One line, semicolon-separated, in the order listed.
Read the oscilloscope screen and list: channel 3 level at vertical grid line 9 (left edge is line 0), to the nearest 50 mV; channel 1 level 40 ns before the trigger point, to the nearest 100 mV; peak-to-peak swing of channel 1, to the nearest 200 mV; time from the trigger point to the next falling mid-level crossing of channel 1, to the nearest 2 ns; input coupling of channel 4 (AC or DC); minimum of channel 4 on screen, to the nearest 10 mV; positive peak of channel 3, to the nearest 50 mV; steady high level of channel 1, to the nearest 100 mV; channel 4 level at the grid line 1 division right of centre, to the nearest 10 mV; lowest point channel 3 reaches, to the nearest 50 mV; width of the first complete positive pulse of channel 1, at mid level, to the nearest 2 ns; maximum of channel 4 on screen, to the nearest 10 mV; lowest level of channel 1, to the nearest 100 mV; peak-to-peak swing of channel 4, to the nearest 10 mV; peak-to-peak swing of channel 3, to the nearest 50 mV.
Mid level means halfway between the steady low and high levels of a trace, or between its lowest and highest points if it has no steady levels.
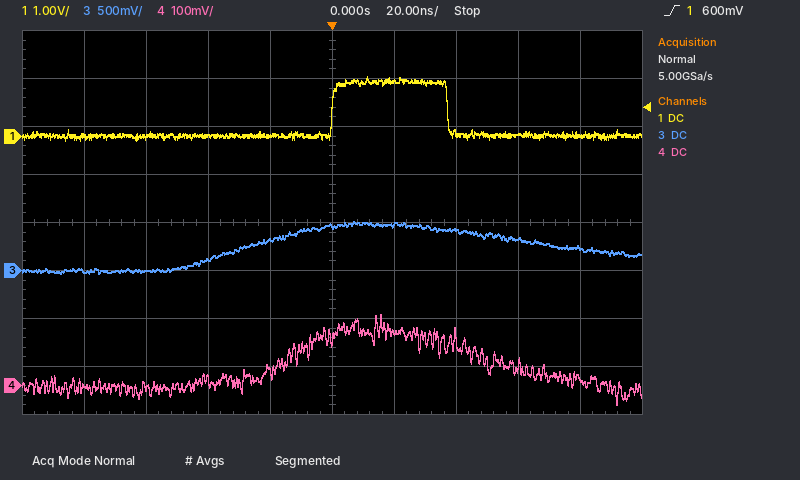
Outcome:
250 mV; 0.0 V; 1.4 V; 38 ns; DC; -40 mV; 500 mV; 1.1 V; 110 mV; -50 mV; 38 ns; 150 mV; -100 mV; 190 mV; 550 mV
